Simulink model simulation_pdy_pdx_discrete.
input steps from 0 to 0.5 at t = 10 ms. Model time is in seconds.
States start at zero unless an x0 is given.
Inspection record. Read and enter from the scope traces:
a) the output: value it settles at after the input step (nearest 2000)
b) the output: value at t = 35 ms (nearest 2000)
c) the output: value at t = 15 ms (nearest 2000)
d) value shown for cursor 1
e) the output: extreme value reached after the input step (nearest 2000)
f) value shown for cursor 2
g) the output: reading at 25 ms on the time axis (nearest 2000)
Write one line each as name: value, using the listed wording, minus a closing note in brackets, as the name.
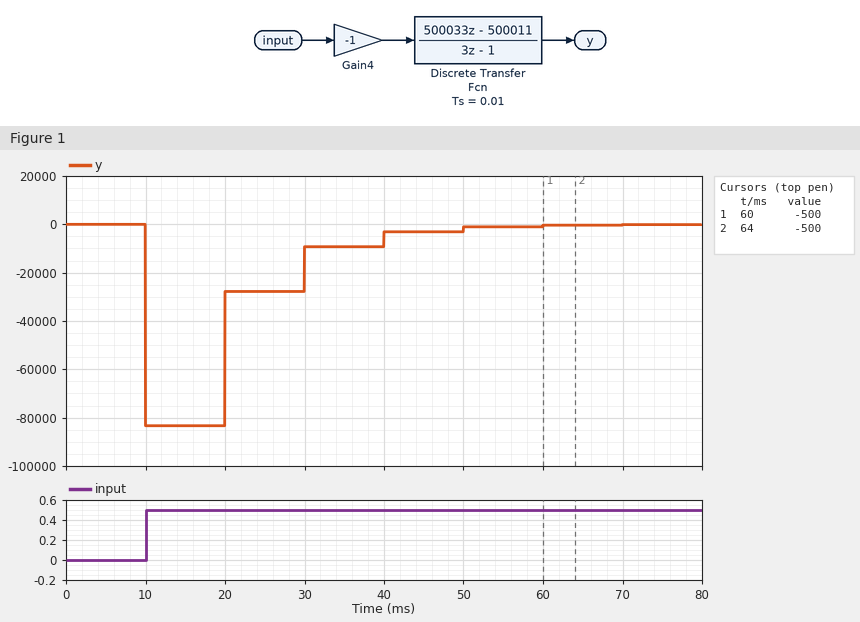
the output: value it settles at after the input step: 0
the output: value at t = 35 ms: -10000
the output: value at t = 15 ms: -84000
value shown for cursor 1: -500
the output: extreme value reached after the input step: -84000
value shown for cursor 2: -500
the output: reading at 25 ms on the time axis: -28000
